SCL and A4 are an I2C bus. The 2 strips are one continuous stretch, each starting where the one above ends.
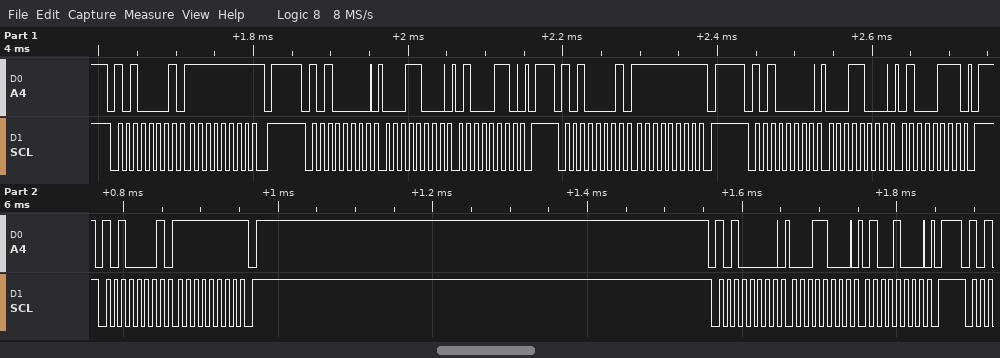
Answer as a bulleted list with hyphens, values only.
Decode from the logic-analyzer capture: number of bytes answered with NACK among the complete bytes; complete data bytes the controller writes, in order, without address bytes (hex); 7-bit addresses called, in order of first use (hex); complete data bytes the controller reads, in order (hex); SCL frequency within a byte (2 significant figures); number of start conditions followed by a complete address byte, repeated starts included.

- 3
- 18 46 18 47 18 48
- 0x50
- FF FF FF
- 100 kHz
- 6
